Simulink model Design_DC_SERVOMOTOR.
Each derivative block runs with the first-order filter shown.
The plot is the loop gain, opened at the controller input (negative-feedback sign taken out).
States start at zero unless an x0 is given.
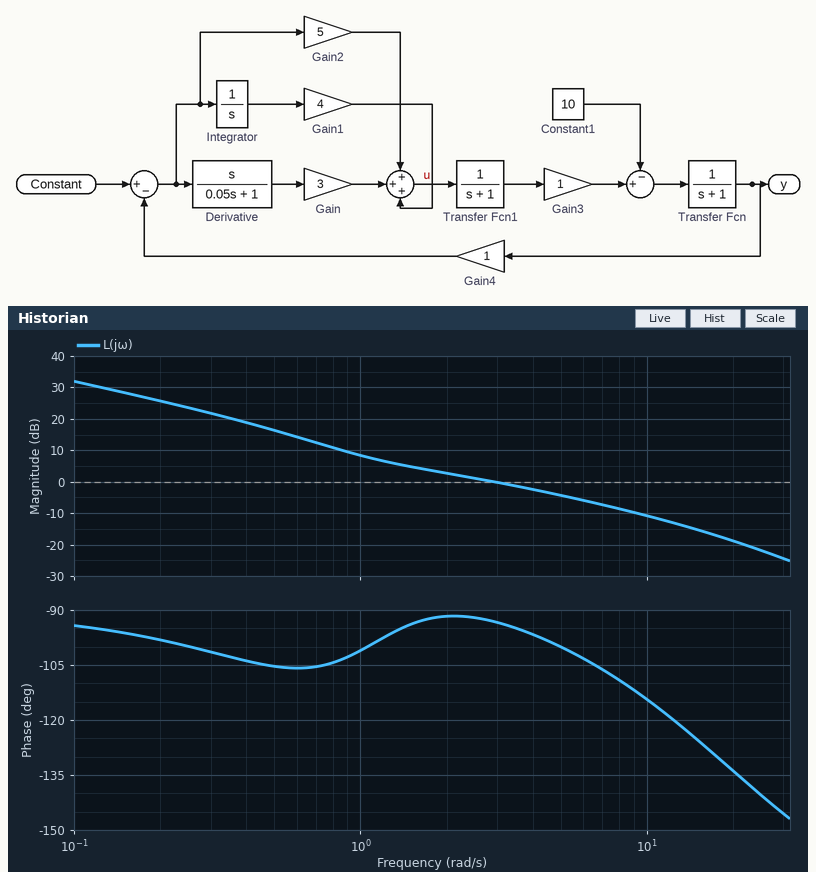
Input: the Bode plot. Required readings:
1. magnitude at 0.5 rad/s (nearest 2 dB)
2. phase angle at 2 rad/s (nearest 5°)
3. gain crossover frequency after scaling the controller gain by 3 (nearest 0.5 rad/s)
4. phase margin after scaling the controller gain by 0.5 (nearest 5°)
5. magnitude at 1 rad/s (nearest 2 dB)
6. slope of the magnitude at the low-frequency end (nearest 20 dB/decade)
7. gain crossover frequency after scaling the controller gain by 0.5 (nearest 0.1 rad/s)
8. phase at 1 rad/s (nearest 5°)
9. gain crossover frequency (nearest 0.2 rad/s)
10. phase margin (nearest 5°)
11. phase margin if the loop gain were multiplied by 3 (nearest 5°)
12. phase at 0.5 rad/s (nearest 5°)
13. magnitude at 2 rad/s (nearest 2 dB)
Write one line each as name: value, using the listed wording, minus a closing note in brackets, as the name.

magnitude at 0.5 rad/s: 16 dB
phase angle at 2 rad/s: -90°
gain crossover frequency after scaling the controller gain by 3: 9.0 rad/s
phase margin after scaling the controller gain by 0.5: 85°
magnitude at 1 rad/s: 8 dB
slope of the magnitude at the low-frequency end: -20 dB/decade
gain crossover frequency after scaling the controller gain by 0.5: 1.3 rad/s
phase at 1 rad/s: -100°
gain crossover frequency: 3.0 rad/s
phase margin: 85°
phase margin if the loop gain were multiplied by 3: 70°
phase at 0.5 rad/s: -105°
magnitude at 2 rad/s: 2 dB
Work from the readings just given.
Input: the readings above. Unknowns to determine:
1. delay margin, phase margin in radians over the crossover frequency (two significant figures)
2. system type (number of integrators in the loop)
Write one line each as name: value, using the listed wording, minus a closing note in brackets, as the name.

delay margin, phase margin in radians over the crossover frequency: 0.49 s
system type: 1
